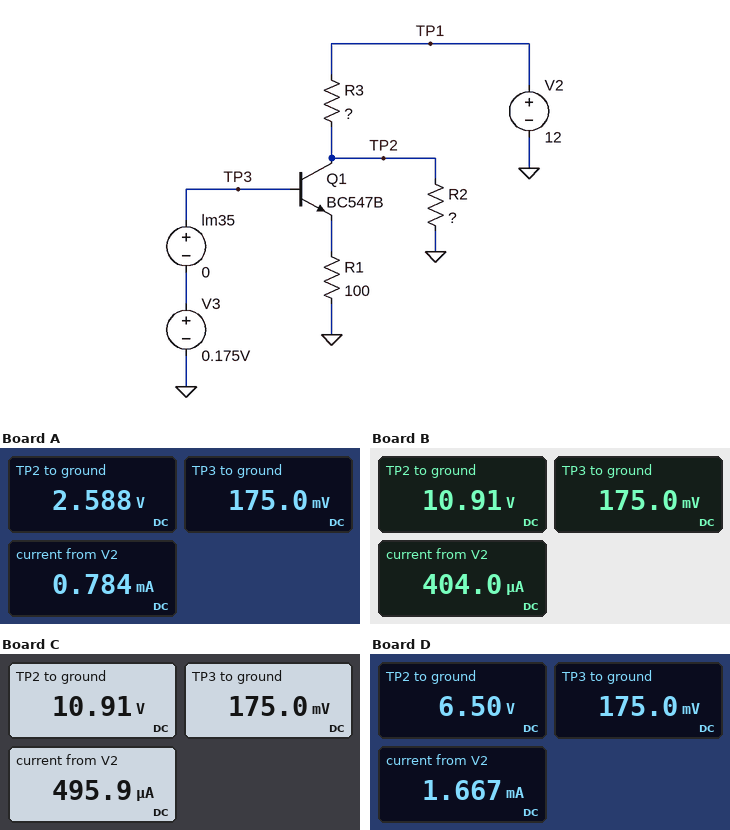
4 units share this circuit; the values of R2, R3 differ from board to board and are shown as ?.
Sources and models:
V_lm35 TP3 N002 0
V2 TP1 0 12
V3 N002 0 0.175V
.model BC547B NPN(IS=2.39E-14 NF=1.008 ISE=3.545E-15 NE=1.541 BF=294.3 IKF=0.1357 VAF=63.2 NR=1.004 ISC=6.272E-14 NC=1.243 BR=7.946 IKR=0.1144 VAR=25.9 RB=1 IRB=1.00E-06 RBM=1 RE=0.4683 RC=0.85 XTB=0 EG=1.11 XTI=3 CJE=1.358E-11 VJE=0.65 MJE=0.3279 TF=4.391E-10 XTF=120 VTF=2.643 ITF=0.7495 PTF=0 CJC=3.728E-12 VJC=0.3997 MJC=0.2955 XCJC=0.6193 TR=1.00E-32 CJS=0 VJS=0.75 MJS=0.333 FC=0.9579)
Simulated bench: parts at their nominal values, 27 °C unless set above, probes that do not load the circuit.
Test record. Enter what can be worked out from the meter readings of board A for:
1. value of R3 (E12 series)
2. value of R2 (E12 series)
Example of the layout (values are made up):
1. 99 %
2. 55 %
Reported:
1. 12 kΩ
2. 3.3 kΩ
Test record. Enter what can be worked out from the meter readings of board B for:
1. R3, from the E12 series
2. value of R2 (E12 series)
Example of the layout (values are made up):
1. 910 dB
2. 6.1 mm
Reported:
1. 2.7 kΩ
2. 27 kΩ
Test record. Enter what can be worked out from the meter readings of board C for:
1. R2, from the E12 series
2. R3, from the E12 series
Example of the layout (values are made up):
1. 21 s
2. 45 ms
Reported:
1. 22 kΩ
2. 2.2 kΩ
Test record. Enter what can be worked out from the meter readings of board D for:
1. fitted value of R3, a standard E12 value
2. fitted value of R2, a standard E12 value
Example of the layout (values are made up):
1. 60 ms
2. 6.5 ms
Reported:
1. 3.3 kΩ
2. 3.9 kΩ
